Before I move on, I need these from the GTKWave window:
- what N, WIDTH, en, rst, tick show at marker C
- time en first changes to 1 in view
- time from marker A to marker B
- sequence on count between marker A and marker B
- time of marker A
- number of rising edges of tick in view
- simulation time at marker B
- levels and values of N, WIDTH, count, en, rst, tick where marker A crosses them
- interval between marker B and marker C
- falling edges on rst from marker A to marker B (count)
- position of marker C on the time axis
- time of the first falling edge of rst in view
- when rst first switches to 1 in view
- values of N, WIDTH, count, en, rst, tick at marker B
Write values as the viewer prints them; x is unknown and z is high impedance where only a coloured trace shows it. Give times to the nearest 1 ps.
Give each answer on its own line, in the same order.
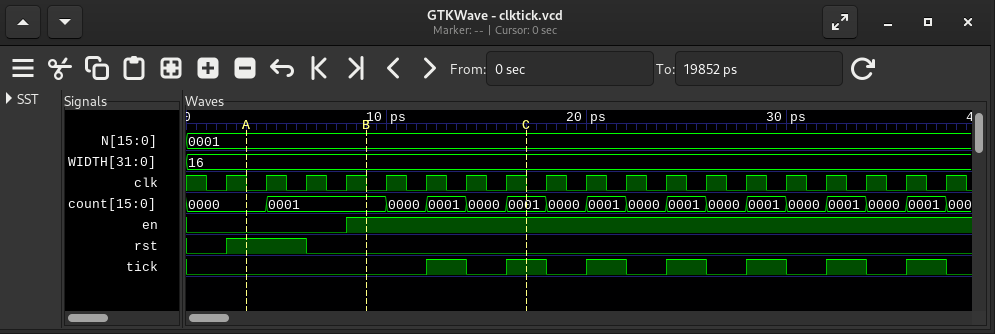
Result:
N=0001, WIDTH=16, en=1, rst=0, tick=1
8 ps
6 ps
0000, 0001
3 ps
7
9 ps
N=0001, WIDTH=16, count=0000, en=0, rst=1, tick=0
8 ps
1
17 ps
6 ps
2 ps
N=0001, WIDTH=16, count=0001, en=1, rst=0, tick=0
